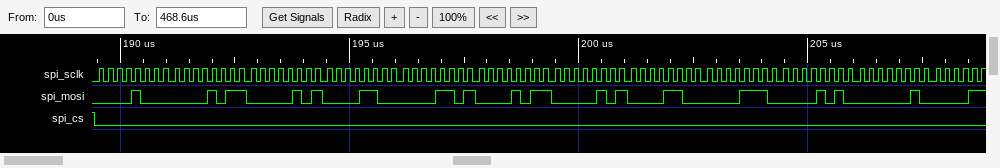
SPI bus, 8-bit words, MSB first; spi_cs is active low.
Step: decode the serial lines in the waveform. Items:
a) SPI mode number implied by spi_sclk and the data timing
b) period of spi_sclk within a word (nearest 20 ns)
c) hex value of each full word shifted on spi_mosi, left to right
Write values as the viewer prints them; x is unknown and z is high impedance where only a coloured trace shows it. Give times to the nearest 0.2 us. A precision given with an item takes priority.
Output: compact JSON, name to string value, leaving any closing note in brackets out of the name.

{"SPI mode number implied by spi_sclk and the data timing": "0", "period of spi_sclk within a word": "200 ns", "hex value of each full word shifted on spi_mosi, left to right": "08, 0B, 05, 0C, 0D, 0B, 05, 0C, 0E, 0A, 02"}
